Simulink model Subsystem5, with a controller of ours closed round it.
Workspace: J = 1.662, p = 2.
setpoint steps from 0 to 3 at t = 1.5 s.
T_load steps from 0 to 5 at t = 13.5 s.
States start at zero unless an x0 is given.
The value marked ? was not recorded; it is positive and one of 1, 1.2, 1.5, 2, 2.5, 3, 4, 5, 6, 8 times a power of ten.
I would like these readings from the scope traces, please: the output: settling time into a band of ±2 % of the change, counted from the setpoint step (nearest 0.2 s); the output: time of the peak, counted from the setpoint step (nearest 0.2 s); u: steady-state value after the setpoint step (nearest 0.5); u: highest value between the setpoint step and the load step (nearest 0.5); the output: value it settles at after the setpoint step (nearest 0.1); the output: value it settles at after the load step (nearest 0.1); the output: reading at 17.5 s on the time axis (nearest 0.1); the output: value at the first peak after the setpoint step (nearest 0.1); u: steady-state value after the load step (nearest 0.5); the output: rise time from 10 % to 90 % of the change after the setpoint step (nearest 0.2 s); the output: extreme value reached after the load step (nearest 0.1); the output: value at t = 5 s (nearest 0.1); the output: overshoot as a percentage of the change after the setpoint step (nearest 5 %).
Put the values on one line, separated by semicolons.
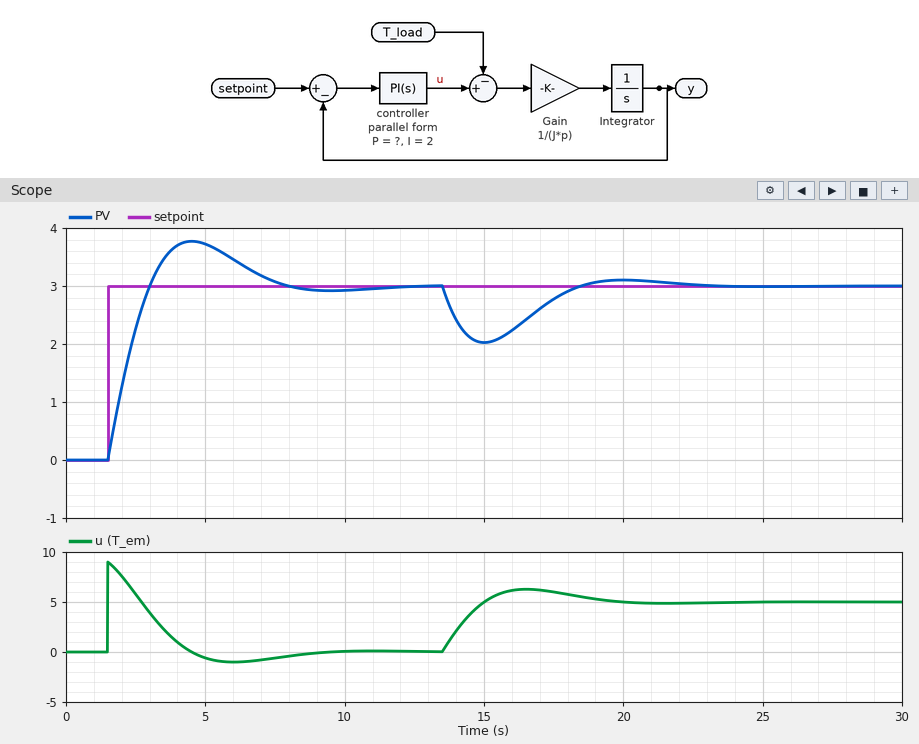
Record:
9.2 s; 3.0 s; 0.0; 9.0; 3.0; 3.0; 2.8; 3.8; 5.0; 1.2 s; 2.0; 3.7; 25 %
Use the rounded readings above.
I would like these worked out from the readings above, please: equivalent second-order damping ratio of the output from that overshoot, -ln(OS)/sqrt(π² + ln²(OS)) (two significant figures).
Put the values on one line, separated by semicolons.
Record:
0.40
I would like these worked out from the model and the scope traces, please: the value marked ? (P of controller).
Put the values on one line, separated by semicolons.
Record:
3
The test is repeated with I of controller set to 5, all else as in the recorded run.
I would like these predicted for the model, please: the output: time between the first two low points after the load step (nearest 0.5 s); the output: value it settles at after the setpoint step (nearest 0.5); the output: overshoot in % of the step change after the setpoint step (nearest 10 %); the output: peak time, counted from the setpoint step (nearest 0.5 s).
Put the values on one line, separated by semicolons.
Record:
5.5 s; 3.0; 40 %; 2.0 s
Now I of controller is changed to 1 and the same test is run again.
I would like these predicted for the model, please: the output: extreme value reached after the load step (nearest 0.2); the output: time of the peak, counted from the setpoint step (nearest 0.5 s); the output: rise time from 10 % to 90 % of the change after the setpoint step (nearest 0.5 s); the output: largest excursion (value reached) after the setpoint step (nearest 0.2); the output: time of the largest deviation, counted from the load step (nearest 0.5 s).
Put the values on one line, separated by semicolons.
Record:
1.8; 4.0 s; 1.5 s; 3.6; 2.0 s
